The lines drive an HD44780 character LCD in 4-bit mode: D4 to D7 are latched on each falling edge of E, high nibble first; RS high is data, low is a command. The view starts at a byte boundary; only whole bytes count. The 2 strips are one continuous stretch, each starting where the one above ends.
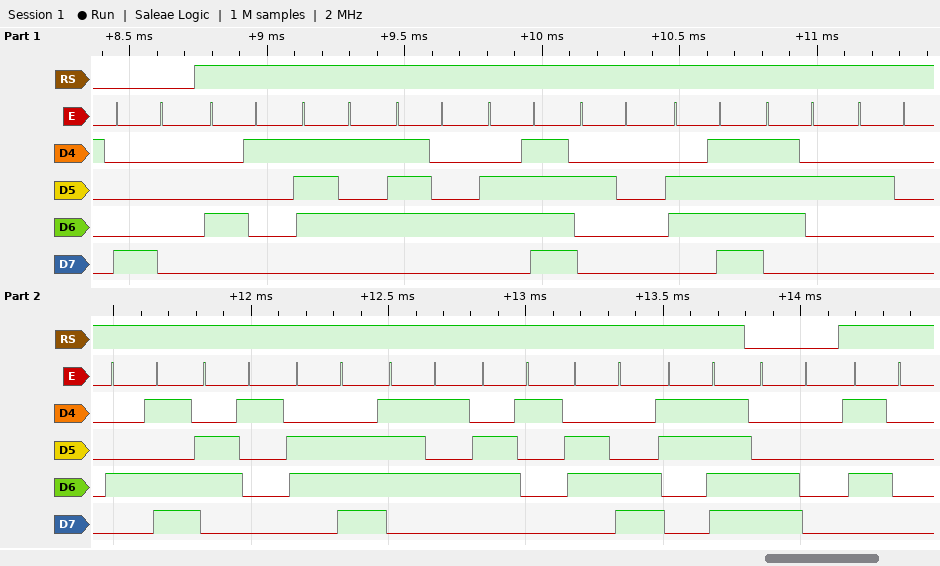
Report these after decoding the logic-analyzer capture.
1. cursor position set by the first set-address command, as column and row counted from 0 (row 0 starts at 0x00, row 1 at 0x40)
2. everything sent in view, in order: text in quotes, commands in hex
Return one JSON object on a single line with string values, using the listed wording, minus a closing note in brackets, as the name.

{"cursor position set by the first set-address command, as column and row counted from 0": "column 0, row 0", "everything sent in view, in order: text in quotes, commands in hex": "0x80 \"Auto or Manual?\" 0xC0 \"P\""}
